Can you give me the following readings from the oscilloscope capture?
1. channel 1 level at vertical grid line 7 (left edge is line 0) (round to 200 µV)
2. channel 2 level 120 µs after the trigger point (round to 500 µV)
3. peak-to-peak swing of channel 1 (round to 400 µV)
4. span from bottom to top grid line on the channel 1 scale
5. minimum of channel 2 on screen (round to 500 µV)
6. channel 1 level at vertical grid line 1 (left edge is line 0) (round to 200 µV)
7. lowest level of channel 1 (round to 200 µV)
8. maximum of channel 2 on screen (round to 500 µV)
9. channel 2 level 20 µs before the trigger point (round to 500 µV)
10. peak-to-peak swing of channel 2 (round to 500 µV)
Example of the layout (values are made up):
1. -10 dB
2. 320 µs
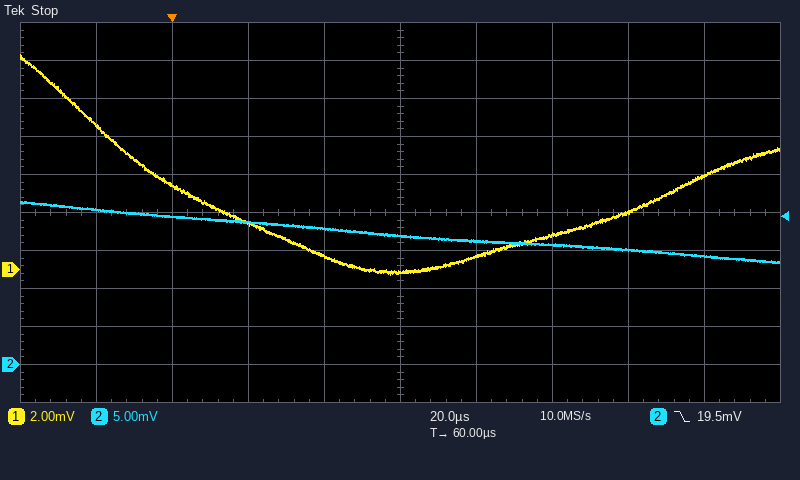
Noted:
1. 1.8 mV
2. 15.0 mV
3. 11.6 mV
4. 20 mV
5. 13.5 mV
6. 7.6 mV
7. -200 µV
8. 21.5 mV
9. 20.5 mV
10. 8.0 mV
